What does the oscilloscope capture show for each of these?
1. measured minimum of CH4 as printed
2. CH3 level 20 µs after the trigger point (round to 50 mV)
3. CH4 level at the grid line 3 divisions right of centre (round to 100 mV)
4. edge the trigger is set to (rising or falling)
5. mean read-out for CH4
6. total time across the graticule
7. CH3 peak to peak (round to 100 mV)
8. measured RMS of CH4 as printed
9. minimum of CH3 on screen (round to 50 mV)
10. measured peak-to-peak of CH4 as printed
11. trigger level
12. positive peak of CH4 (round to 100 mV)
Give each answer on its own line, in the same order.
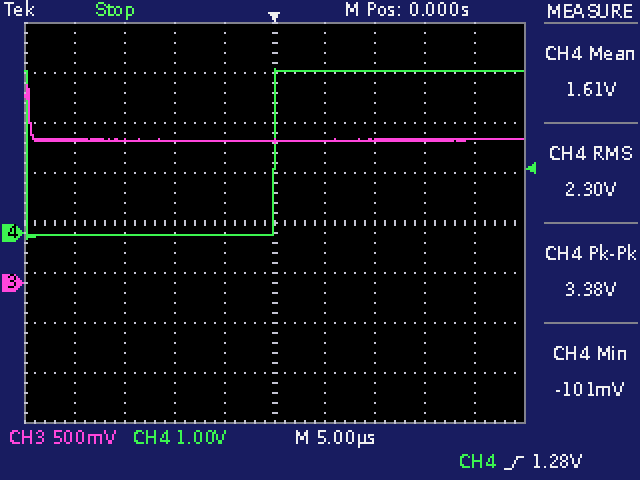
-101 mV
1.45 V
3.2 V
rising
1.61 V
50 µs
600 mV
2.30 V
1.40 V
3.38 V
1.28 V
3.3 V
